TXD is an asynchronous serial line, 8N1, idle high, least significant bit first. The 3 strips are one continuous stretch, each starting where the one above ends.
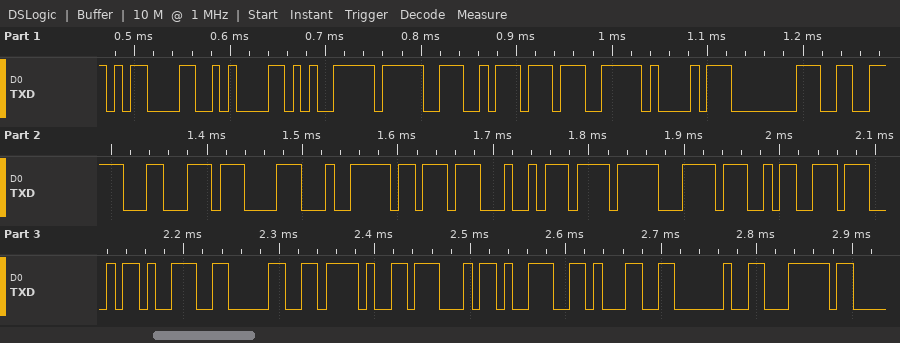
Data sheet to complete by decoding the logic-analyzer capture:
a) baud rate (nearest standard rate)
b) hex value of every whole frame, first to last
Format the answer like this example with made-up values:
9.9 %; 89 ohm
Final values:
115200 baud; 0D 0A E5 9F BA E7 A1 80 E6 8C 87 E4 BB A4 EF BC 9A 47 39 30 2F 47 39 31 20 7C
